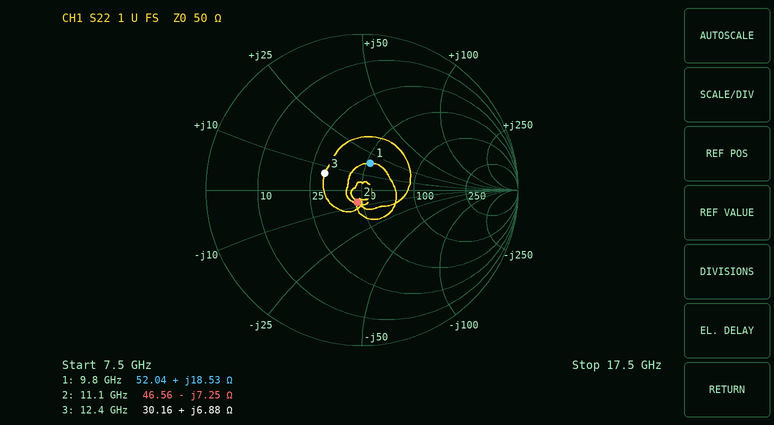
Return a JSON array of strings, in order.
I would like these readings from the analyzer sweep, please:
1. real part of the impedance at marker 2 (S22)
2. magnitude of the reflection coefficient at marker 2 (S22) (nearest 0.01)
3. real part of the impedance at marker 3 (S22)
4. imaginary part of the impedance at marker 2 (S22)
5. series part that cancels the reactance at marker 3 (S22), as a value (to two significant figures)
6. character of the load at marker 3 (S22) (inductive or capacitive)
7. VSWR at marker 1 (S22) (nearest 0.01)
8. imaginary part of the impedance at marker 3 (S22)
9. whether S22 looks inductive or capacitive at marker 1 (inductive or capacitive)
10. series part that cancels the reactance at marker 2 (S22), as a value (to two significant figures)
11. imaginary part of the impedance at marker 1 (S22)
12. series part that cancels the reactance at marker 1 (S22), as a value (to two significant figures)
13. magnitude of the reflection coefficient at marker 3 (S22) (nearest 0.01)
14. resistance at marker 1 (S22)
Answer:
["46.56 Ω", "0.08", "30.16 Ω", "-7.25 Ω", "1.9 pF", "inductive", "1.44", "+6.88 Ω", "inductive", "100 pH", "+18.53 Ω", "880 fF", "0.26", "52.04 Ω"]
